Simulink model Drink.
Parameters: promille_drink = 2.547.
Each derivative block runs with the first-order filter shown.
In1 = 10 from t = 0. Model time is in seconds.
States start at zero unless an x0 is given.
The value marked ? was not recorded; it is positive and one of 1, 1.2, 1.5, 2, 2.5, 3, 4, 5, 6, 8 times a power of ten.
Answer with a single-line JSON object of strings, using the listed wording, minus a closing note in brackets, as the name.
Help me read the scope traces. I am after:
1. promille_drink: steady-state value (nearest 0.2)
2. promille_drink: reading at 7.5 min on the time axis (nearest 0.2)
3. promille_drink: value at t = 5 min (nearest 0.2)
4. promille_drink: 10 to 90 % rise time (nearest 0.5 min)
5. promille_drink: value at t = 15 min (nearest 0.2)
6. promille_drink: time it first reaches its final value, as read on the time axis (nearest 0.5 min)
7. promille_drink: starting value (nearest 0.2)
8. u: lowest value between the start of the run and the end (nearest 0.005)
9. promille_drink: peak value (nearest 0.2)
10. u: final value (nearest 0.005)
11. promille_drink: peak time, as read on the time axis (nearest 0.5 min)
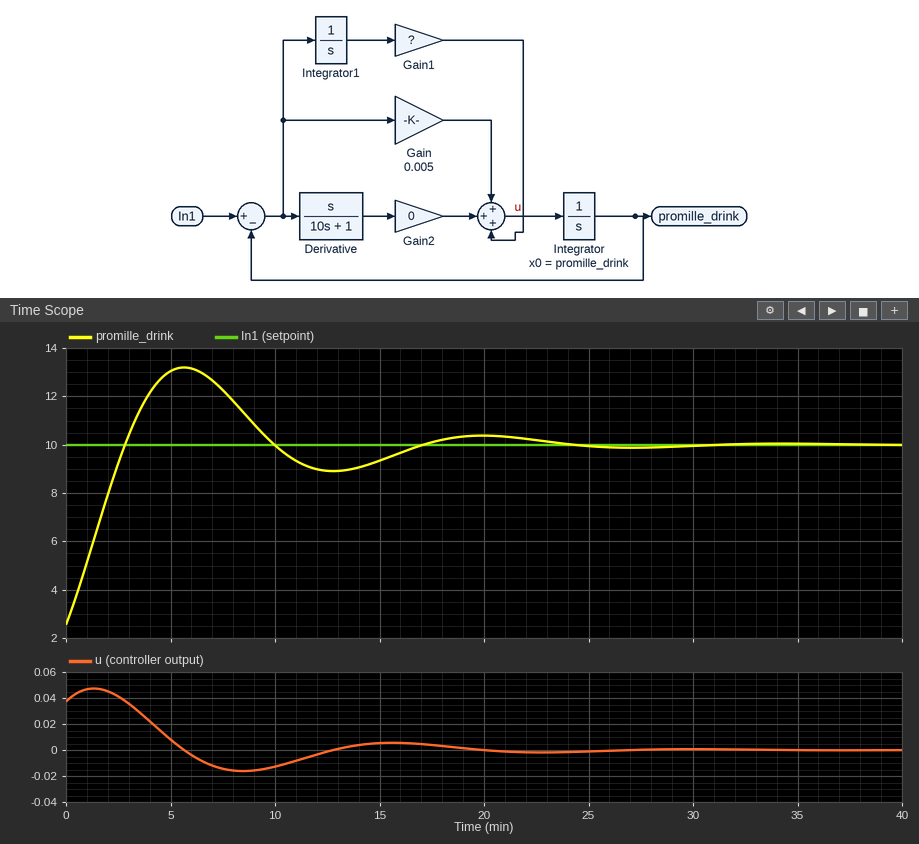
{"promille_drink: steady-state value": "10.0", "promille_drink: reading at 7.5 min on the time axis": "12.2", "promille_drink: value at t = 5 min": "13.0", "promille_drink: 10 to 90 % rise time": "2.0 min", "promille_drink: value at t = 15 min": "9.4", "promille_drink: time it first reaches its final value, as read on the time axis": "3.0 min", "promille_drink: starting value": "2.6", "u: lowest value between the start of the run and the end": "-0.015", "promille_drink: peak value": "13.2", "u: final value": "0.000", "promille_drink: peak time, as read on the time axis": "5.5 min"}
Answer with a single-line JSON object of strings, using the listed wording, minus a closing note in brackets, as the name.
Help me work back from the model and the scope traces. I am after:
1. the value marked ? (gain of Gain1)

{"the value marked ?": "6e-05"}
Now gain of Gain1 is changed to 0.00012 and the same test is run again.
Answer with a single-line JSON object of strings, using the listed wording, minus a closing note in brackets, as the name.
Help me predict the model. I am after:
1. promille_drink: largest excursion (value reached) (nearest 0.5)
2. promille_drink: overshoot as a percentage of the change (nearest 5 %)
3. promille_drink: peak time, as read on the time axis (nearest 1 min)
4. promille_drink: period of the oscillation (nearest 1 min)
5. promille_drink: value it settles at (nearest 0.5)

{"promille_drink: largest excursion (value reached)": "14.0", "promille_drink: overshoot as a percentage of the change": "55 %", "promille_drink: peak time, as read on the time axis": "4 min", "promille_drink: period of the oscillation": "10 min", "promille_drink: value it settles at": "10.0"}
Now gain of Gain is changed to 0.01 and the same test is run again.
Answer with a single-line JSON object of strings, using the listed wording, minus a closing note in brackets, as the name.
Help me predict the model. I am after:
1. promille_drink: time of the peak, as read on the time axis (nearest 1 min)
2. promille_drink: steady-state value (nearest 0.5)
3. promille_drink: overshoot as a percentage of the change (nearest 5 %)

{"promille_drink: time of the peak, as read on the time axis": "5 min", "promille_drink: steady-state value": "10.0", "promille_drink: overshoot as a percentage of the change": "25 %"}
